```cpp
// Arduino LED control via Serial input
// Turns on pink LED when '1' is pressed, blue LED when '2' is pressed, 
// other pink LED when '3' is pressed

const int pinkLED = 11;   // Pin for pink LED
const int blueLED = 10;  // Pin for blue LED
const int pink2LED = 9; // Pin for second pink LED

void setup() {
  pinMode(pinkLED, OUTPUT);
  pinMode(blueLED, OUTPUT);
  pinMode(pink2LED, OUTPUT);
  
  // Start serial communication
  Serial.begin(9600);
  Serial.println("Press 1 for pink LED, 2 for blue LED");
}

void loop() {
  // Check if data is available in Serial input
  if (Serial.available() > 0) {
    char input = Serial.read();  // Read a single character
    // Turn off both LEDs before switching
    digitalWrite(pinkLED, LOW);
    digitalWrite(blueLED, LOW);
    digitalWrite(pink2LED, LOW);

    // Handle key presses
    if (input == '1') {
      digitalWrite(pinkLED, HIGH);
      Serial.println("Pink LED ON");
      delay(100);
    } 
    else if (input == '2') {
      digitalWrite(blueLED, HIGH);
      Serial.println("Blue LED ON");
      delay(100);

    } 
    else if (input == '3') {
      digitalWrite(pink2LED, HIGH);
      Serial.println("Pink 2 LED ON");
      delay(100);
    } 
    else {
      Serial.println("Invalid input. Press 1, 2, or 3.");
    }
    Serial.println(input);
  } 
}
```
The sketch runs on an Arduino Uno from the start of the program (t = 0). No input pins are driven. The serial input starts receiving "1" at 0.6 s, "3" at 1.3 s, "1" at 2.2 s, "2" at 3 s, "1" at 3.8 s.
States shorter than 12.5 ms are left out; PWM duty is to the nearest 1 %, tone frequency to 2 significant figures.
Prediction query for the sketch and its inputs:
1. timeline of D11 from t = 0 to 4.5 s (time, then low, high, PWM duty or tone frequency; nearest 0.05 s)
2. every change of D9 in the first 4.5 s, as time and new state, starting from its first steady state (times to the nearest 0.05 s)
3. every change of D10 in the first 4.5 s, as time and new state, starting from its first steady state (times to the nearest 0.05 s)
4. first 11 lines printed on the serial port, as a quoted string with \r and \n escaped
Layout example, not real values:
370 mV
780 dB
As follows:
0 s low; 0.6 s high; 1.3 s low; 2.2 s high; 3 s low; 3.8 s high
0 s low; 1.3 s high; 2.2 s low
0 s low; 3 s high; 3.8 s low
"Press 1 for pink LED, 2 for blue LED\r\nPink LED ON\r\n1\r\nPink 2 LED ON\r\n3\r\nPink LED ON\r\n1\r\nBlue LED ON\r\n2\r\nPink LED ON\r\n1\r\n"
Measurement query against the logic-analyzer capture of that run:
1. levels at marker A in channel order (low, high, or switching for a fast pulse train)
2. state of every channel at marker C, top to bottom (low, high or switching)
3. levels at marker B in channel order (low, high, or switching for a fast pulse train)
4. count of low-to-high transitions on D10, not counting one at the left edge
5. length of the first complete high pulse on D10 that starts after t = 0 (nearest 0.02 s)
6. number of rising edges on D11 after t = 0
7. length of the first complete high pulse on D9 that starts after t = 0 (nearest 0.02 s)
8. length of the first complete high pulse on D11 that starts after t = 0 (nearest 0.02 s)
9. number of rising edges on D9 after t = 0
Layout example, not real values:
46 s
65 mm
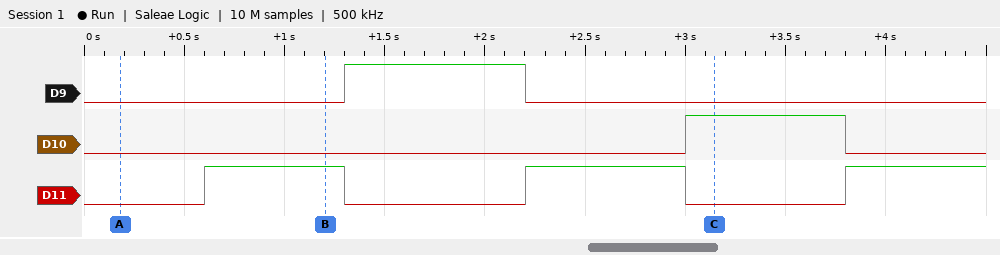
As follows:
D9 low, D10 low, D11 low
D9 low, D10 high, D11 low
D9 low, D10 low, D11 high
1
0.80 s
3
0.90 s
0.70 s
1
